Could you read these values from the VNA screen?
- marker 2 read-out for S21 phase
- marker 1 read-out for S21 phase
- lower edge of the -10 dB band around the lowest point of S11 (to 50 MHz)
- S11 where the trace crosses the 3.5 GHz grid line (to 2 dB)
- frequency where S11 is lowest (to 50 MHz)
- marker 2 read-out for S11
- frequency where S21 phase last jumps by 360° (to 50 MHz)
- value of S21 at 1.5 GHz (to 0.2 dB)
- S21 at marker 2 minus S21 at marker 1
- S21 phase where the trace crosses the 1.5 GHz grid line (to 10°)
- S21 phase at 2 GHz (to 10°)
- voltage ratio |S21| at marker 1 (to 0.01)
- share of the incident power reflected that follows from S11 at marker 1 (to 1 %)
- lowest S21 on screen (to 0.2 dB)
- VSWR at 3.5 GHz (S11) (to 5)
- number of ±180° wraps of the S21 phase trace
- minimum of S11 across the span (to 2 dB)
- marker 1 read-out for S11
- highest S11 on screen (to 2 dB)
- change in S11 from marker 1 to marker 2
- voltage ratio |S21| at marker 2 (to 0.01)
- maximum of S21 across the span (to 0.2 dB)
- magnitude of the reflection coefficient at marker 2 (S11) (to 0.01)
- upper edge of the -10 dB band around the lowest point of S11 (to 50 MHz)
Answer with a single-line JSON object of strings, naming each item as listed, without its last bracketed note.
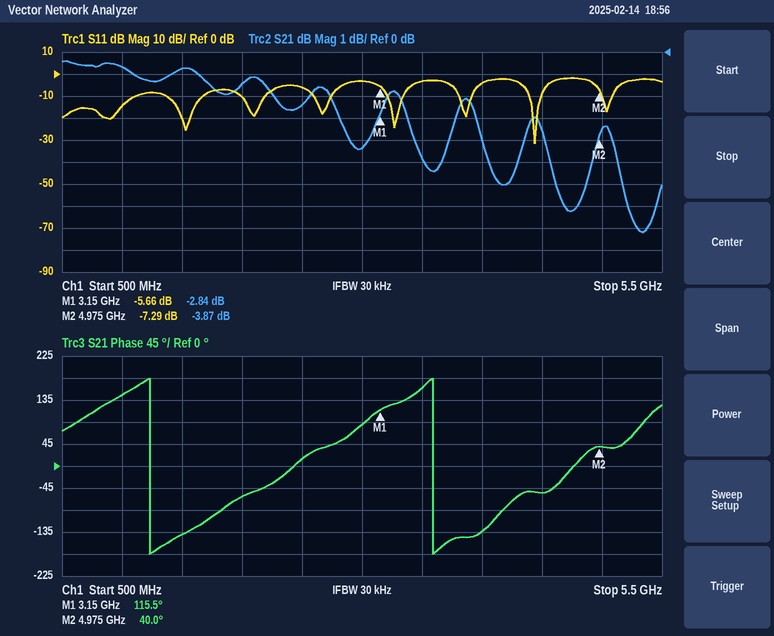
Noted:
{"marker 2 read-out for S21 phase": "40.0°", "marker 1 read-out for S21 phase": "115.5°", "lower edge of the -10 dB band around the lowest point of S11": "4.40 GHz", "S11 where the trace crosses the 3.5 GHz grid line": "-4 dB", "frequency where S11 is lowest": "4.45 GHz", "marker 2 read-out for S11": "-7.29 dB", "frequency where S21 phase last jumps by 360°": "3.60 GHz", "value of S21 at 1.5 GHz": "-0.8 dB", "S21 at marker 2 minus S21 at marker 1": "-1.03 dB", "S21 phase where the trace crosses the 1.5 GHz grid line": "-140°", "S21 phase at 2 GHz": "-60°", "voltage ratio |S21| at marker 1": "0.72", "share of the incident power reflected that follows from S11 at marker 1": "27 %", "lowest S21 on screen": "-8.2 dB", "VSWR at 3.5 GHz (S11)": "5", "number of ±180° wraps of the S21 phase trace": "2", "minimum of S11 across the span": "-32 dB", "marker 1 read-out for S11": "-5.66 dB", "highest S11 on screen": "-2 dB", "change in S11 from marker 1 to marker 2": "-1.63 dB", "voltage ratio |S21| at marker 2": "0.64", "maximum of S21 across the span": "-0.4 dB", "magnitude of the reflection coefficient at marker 2 (S11)": "0.43", "upper edge of the -10 dB band around the lowest point of S11": "4.50 GHz"}
